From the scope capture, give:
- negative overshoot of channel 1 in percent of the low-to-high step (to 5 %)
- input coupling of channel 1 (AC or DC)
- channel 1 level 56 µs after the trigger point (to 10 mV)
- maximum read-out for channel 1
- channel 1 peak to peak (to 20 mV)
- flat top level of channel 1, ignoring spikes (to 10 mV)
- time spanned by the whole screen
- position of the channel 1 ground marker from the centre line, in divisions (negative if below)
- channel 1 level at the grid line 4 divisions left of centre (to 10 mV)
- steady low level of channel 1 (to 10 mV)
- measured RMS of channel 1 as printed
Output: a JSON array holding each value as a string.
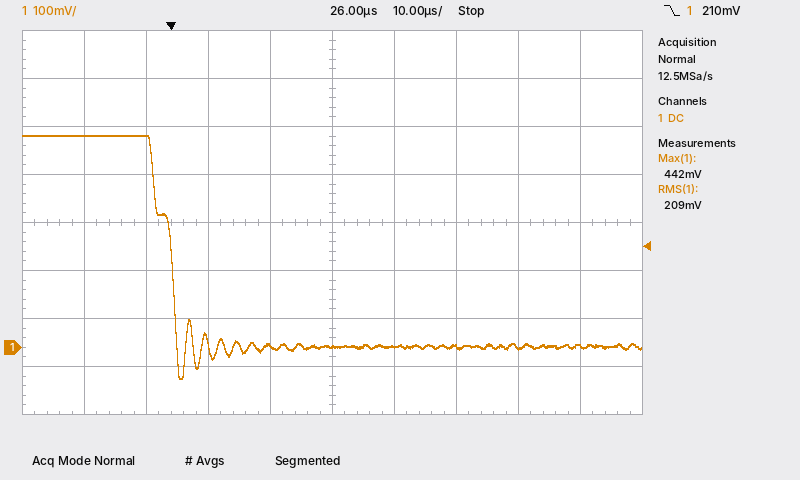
["15 %", "DC", "0 mV", "442 mV", "500 mV", "440 mV", "100 µs", "-2.6 div", "440 mV", "0 mV", "209 mV"]
